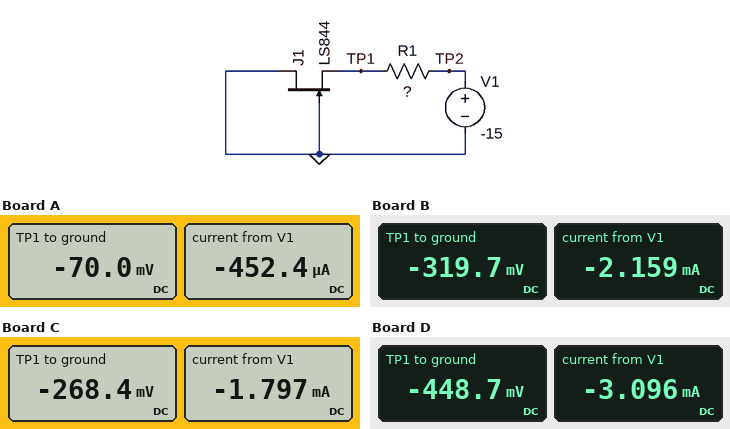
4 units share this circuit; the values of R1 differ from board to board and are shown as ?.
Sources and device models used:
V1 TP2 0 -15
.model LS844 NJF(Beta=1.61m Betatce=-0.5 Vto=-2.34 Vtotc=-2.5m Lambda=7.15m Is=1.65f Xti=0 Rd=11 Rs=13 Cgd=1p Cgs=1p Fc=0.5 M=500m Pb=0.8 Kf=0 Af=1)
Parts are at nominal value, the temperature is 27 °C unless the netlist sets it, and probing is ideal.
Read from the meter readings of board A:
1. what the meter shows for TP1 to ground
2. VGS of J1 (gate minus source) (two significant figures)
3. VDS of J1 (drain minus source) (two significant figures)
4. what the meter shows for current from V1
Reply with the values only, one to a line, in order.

-70.0 mV
70 mV
70 mV
-452.4 µA
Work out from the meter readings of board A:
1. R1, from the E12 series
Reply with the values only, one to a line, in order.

33 kΩ
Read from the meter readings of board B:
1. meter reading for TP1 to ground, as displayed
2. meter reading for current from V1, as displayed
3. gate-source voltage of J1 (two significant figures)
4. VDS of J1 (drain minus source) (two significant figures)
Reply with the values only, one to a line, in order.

-319.7 mV
-2.159 mA
320 mV
320 mV
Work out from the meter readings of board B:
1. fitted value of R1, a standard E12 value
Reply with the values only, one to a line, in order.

6.8 kΩ
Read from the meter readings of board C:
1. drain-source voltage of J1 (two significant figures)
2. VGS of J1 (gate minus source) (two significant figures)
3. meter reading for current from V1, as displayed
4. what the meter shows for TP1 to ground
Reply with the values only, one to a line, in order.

270 mV
270 mV
-1.797 mA
-268.4 mV
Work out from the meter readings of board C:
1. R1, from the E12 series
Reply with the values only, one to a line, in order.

8.2 kΩ
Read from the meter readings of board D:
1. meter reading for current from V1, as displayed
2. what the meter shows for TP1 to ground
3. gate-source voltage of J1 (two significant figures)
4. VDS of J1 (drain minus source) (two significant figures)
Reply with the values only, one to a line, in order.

-3.096 mA
-448.7 mV
450 mV
450 mV
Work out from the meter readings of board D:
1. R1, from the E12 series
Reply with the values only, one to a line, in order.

4.7 kΩ
